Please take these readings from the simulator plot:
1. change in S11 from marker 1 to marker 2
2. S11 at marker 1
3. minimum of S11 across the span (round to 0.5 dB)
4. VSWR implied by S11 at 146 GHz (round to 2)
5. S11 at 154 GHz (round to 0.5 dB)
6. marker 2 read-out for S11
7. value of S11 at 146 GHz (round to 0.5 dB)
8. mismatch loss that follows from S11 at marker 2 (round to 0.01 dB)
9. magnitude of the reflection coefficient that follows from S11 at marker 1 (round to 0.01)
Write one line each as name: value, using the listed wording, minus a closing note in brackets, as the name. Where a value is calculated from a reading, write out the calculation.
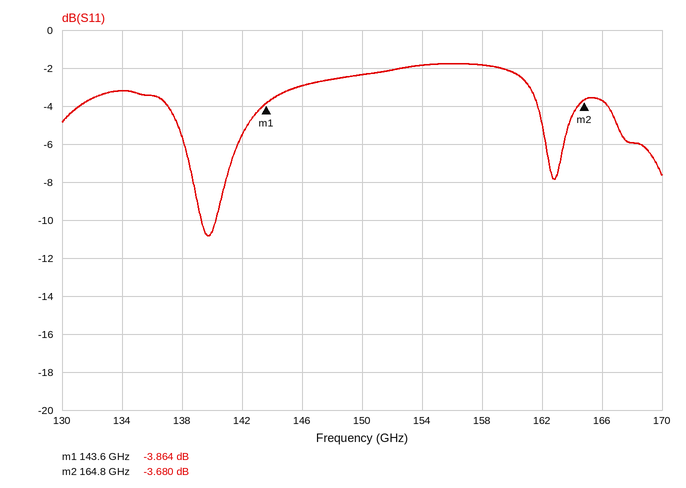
change in S11 from marker 1 to marker 2: -3.68 − (-3.864) = 0.184 dB
S11 at marker 1: -3.864 dB
minimum of S11 across the span: -11.0 dB
VSWR implied by S11 at 146 GHz: |Γ| = 10^(-3/20) = 0.7079; VSWR = (1 + 0.7079)/(1 − 0.7079) ≈ 6
S11 at 154 GHz: -2.0 dB
marker 2 read-out for S11: -3.680 dB
value of S11 at 146 GHz: -3.0 dB
mismatch loss that follows from S11 at marker 2: −10 log10(1 − 10^(-3.68/10)) ≈ 2.43 dB
magnitude of the reflection coefficient that follows from S11 at marker 1: 10^(-3.864/20) ≈ 0.64
